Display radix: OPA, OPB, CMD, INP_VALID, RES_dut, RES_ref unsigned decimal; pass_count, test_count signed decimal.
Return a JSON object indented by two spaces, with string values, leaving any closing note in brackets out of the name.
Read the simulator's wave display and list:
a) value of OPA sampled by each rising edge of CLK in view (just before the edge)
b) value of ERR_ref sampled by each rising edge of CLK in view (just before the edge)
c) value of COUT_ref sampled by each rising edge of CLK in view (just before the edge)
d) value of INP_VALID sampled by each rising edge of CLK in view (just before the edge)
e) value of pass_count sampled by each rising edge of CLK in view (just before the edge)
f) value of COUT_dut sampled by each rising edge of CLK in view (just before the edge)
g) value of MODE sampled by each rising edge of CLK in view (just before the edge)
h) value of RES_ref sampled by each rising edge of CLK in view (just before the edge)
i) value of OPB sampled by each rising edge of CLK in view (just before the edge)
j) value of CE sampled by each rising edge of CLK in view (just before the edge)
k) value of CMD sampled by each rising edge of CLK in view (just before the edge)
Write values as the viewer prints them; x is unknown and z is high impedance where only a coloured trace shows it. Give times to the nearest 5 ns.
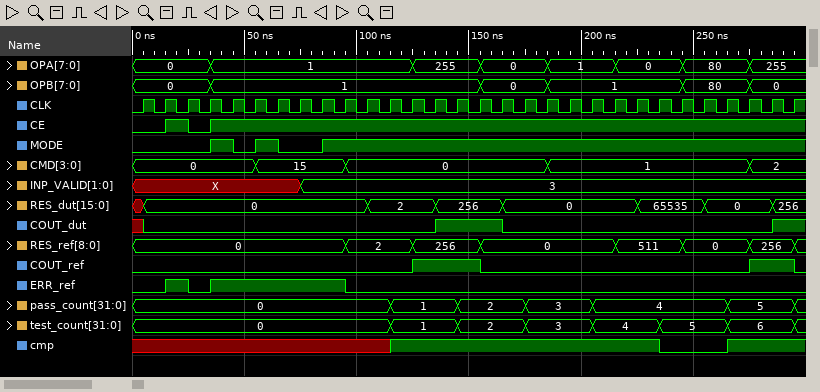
{
  "value of OPA sampled by each rising edge of CLK in view": "0, 0, 0, 0, 1, 1, 1, 1, 1, 1, 1, 1, 1, 255, 255, 255, 0, 0, 0, 1, 1, 1, 0, 0, 0, 80, 80, 80, 255, 255",
  "value of ERR_ref sampled by each rising edge of CLK in view": "0 0 1 0 1 1 1 1 1 1 0 0 0 0 0 0 0 0 0 0 0 0 0 0 0 0 0 0 0 0",
  "value of COUT_ref sampled by each rising edge of CLK in view": "0 0 0 0 0 0 0 0 0 0 0 0 0 1 1 1 0 0 0 0 0 0 0 0 0 0 0 0 1 1",
  "value of INP_VALID sampled by each rising edge of CLK in view": "X, X, X, X, X, X, X, X, 3, 3, 3, 3, 3, 3, 3, 3, 3, 3, 3, 3, 3, 3, 3, 3, 3, 3, 3, 3, 3, 3",
  "value of pass_count sampled by each rising edge of CLK in view": "0, 0, 0, 0, 0, 0, 0, 0, 0, 0, 0, 0, 1, 1, 1, 2, 2, 2, 3, 3, 3, 4, 4, 4, 4, 4, 4, 5, 5, 5",
  "value of COUT_dut sampled by each rising edge of CLK in view": "x 0 0 0 0 0 0 0 0 0 0 0 0 0 1 1 1 0 0 0 0 0 0 0 0 0 0 0 0 1",
  "value of MODE sampled by each rising edge of CLK in view": "0 0 0 0 1 0 1 0 0 1 1 1 1 1 1 1 1 1 1 1 1 1 1 1 1 1 1 1 1 1",
  "value of RES_ref sampled by each rising edge of CLK in view": "0, 0, 0, 0, 0, 0, 0, 0, 0, 0, 2, 2, 2, 256, 256, 256, 0, 0, 0, 0, 0, 0, 511, 511, 511, 0, 0, 0, 256, 256",
  "value of OPB sampled by each rising edge of CLK in view": "0, 0, 0, 0, 1, 1, 1, 1, 1, 1, 1, 1, 1, 1, 1, 1, 0, 0, 0, 1, 1, 1, 1, 1, 1, 80, 80, 80, 0, 0",
  "value of CE sampled by each rising edge of CLK in view": "0 0 1 0 1 1 1 1 1 1 1 1 1 1 1 1 1 1 1 1 1 1 1 1 1 1 1 1 1 1",
  "value of CMD sampled by each rising edge of CLK in view": "0, 0, 0, 0, 0, 0, 15, 15, 15, 15, 0, 0, 0, 0, 0, 0, 0, 0, 0, 1, 1, 1, 1, 1, 1, 1, 1, 1, 2, 2"
}
